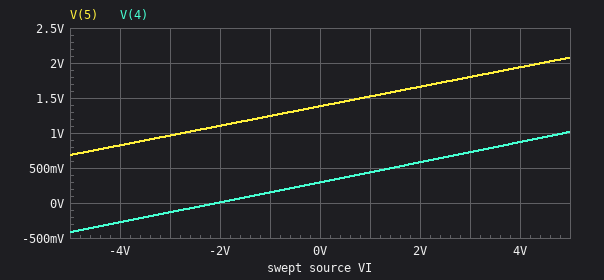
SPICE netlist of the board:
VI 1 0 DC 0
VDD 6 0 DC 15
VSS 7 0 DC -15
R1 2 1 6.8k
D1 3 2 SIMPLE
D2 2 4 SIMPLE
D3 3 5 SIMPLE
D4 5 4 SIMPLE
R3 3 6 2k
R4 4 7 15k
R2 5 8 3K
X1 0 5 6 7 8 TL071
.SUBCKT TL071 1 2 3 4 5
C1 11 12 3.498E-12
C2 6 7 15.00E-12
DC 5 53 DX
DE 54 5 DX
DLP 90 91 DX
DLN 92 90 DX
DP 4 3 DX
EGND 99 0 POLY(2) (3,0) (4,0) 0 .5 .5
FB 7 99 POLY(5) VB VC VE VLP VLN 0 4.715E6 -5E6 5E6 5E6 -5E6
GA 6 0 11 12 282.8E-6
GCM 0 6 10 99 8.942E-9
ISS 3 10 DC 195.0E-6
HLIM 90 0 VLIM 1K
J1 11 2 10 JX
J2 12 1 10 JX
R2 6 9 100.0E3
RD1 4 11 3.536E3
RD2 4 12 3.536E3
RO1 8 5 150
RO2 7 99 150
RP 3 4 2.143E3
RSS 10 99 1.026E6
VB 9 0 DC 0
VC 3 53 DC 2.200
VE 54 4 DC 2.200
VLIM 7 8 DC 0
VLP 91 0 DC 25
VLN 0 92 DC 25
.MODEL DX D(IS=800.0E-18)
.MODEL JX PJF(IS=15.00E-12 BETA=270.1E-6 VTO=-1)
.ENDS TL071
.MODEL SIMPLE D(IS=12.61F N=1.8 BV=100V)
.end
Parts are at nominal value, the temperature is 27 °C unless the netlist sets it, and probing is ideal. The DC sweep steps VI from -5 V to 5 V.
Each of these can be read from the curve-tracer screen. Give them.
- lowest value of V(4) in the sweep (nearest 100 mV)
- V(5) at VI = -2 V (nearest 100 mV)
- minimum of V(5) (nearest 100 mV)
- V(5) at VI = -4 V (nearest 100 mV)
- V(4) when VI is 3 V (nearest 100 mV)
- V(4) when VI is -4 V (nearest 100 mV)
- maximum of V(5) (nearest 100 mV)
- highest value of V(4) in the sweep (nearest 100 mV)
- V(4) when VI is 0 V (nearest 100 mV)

-400 mV
1.1 V
700 mV
800 mV
700 mV
-300 mV
2.1 V
1.0 V
300 mV
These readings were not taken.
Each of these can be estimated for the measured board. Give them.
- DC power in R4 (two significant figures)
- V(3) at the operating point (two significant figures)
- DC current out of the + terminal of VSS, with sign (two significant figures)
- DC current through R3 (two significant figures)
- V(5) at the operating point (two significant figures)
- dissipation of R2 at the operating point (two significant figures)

16 mW
2.6 V
-15 mA
6.2 mA
1.4 V
74 mW
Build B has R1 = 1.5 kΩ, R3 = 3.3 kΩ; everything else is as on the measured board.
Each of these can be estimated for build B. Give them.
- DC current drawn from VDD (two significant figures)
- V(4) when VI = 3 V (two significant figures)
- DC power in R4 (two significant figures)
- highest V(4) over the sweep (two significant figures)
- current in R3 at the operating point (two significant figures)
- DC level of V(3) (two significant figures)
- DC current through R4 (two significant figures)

18 mA
300 mV
13 mW
2.1 V
4.2 mA
1.2 V
930 µA
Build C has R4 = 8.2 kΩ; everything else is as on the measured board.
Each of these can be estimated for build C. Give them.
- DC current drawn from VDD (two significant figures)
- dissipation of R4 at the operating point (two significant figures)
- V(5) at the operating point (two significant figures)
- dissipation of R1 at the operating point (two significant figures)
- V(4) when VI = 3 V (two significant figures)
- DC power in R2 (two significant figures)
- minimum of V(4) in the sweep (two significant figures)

21 mA
26 mW
620 mV
68 µW
-99 mV
66 mW
-1.1 V
